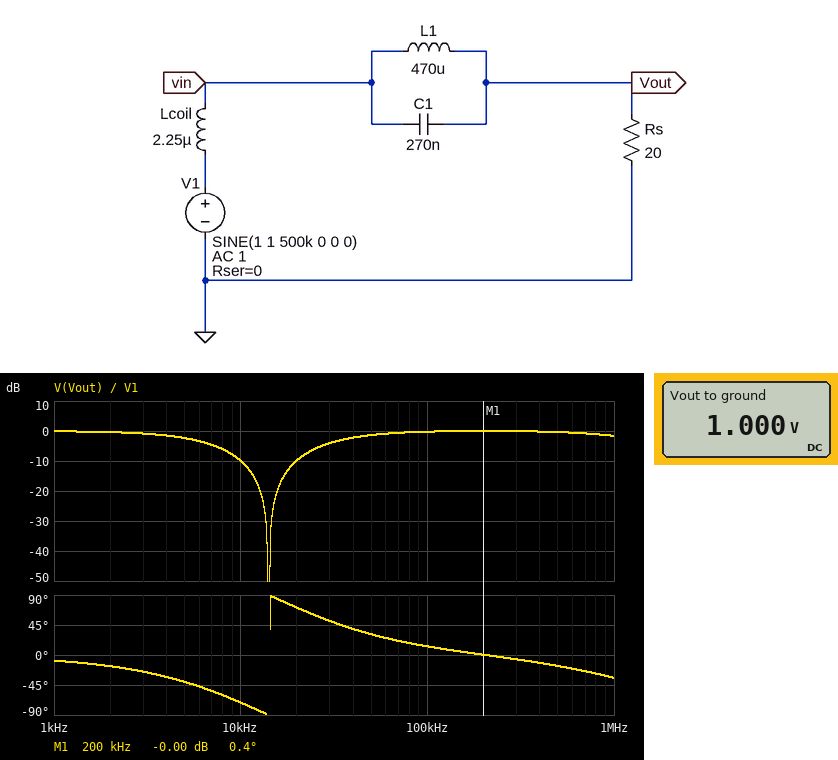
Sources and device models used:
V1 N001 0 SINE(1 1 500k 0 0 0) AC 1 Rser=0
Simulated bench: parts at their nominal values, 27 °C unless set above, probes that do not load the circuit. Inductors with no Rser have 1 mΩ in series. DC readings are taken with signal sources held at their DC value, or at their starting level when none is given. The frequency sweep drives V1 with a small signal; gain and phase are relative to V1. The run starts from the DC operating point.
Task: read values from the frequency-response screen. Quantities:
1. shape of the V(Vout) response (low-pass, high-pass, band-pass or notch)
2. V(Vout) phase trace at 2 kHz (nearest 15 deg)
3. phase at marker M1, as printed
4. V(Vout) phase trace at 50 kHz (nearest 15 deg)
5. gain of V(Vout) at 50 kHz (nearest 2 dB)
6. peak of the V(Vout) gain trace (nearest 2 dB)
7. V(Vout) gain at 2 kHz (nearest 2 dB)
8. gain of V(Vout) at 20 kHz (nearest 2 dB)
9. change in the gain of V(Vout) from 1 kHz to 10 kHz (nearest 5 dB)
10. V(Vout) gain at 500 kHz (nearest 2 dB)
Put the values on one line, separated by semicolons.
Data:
notch; -15 deg; 0.4 deg; 30 deg; -2 dB; 0 dB; 0 dB; -10 dB; -10 dB; 0 dB
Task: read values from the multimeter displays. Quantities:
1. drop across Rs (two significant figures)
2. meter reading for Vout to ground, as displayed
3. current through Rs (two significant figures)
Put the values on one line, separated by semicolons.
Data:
1.0 V; 1.000 V; 50 mA
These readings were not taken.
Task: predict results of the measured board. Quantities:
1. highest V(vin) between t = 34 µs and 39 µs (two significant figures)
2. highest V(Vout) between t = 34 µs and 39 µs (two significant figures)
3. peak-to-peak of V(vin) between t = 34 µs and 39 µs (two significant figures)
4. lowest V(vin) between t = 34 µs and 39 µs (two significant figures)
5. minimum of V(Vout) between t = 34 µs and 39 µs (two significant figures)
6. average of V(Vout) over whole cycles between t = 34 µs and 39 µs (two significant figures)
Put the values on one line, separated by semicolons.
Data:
2.0 V; 2.0 V; 1.9 V; 39 mV; 45 mV; 1.0 V
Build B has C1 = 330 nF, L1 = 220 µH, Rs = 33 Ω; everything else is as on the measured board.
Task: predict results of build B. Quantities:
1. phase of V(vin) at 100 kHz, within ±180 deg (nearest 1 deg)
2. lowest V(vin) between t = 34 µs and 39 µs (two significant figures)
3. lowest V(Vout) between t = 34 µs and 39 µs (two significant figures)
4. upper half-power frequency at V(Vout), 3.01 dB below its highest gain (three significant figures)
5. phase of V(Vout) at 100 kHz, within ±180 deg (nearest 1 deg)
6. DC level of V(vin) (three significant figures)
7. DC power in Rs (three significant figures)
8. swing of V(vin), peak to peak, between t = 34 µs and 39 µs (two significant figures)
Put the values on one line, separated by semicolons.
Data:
-2 deg; 16 mV; 18 mV; 2.35 MHz; 6 deg; 1.00 V; 30.3 mW; 2.0 V
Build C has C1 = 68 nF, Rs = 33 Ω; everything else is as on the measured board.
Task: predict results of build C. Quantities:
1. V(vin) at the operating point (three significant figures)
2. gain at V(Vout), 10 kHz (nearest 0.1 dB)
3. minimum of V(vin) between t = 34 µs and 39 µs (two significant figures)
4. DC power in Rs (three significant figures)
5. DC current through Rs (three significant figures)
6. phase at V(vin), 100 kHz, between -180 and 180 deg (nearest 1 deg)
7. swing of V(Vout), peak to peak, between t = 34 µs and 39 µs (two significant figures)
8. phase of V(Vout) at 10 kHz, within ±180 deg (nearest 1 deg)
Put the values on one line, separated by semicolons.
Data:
1.00 V; -3.1 dB; -7.5 mV; 30.3 mW; 30.3 mA; -2 deg; 2.0 V; -46 deg
